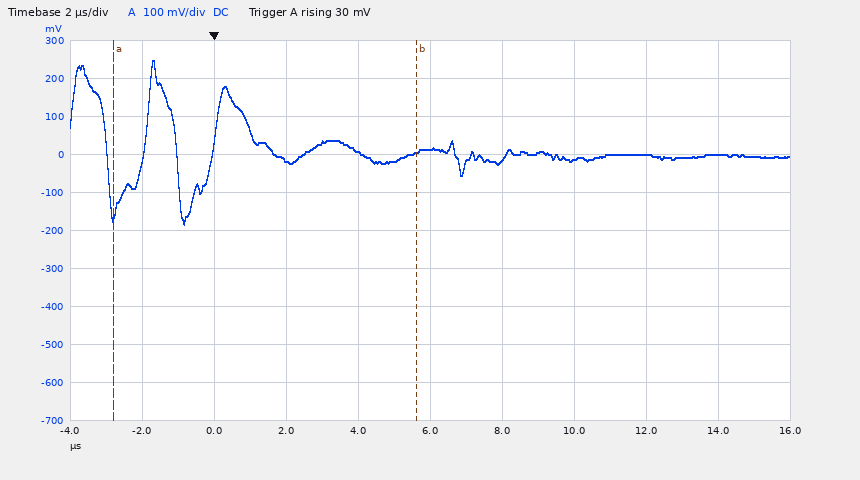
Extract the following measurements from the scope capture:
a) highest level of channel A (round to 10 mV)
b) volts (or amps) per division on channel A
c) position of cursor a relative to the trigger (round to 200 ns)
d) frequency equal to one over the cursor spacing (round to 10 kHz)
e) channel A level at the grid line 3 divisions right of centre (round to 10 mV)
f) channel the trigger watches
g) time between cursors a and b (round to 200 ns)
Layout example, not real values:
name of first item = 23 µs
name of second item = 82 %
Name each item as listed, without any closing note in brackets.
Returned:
highest level of channel A = 250 mV
volts (or amps) per division on channel A = 100 mV
position of cursor a relative to the trigger = -2.8 µs
frequency equal to one over the cursor spacing = 120 kHz
channel A level at the grid line 3 divisions right of centre = 0 mV
channel the trigger watches = channel A
time between cursors a and b = 8.4 µs
